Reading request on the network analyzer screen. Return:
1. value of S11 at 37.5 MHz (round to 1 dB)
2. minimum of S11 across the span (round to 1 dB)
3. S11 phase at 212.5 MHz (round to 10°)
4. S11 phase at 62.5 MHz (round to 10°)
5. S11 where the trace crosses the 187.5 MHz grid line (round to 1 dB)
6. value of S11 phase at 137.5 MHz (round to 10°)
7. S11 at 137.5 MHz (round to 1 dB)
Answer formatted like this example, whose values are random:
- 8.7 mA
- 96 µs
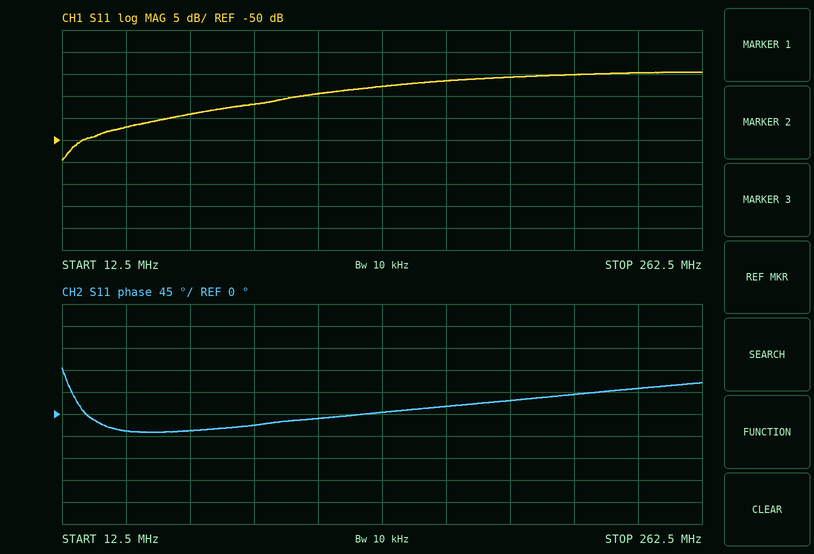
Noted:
- -47 dB
- -55 dB
- 40°
- -30°
- -36 dB
- 0°
- -38 dB
